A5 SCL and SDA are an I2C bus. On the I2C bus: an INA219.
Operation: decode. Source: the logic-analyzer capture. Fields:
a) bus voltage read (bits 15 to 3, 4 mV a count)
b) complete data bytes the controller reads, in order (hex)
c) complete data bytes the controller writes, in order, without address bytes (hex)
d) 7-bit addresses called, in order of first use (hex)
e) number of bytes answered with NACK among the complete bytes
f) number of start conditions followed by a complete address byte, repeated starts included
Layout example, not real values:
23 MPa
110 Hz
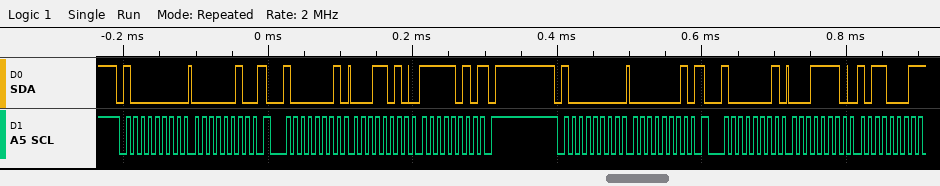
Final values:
3.452 V
1A FA 1E B1
02 01
0x40
2
4
